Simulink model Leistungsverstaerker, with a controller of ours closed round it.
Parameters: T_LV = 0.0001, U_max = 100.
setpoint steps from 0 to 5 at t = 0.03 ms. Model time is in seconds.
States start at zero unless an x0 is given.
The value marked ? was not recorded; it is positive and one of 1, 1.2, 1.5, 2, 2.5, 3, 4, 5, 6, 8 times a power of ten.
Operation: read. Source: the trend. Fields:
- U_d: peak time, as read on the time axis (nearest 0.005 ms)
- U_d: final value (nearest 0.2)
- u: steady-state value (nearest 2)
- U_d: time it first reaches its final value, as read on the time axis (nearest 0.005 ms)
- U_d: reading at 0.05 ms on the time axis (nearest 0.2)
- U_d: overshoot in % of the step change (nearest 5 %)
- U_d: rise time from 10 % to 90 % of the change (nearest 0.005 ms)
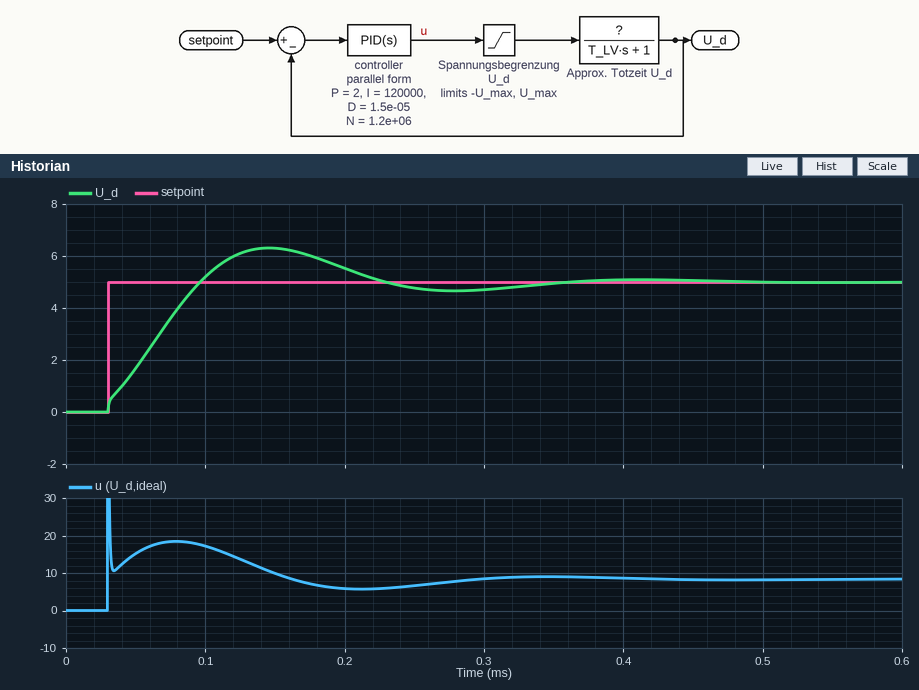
0.145 ms
5.0
8
0.095 ms
1.6
25 %
0.055 ms
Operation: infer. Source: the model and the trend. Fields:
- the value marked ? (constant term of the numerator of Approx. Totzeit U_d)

0.6
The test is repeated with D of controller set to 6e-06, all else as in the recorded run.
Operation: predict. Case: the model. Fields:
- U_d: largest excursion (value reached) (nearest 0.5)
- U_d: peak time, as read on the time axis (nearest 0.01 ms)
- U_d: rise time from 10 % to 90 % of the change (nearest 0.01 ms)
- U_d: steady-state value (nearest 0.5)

6.5
0.14 ms
0.05 ms
5.0
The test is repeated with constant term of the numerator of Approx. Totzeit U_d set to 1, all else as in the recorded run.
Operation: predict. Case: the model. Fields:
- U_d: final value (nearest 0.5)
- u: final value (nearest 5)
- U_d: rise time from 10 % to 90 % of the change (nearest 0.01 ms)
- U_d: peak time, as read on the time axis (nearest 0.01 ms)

5.0
5
0.04 ms
0.12 ms
